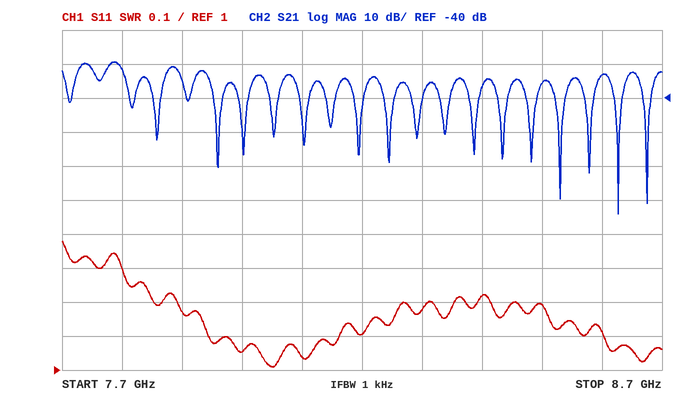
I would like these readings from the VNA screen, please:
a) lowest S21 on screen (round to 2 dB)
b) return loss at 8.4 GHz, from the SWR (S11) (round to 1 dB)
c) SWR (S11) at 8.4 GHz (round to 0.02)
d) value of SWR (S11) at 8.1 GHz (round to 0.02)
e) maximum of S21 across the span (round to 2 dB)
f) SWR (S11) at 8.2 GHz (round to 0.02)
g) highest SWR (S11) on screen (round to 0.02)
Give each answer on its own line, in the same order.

-74 dB
20 dB
1.22
1.04
-30 dB
1.10
1.38
